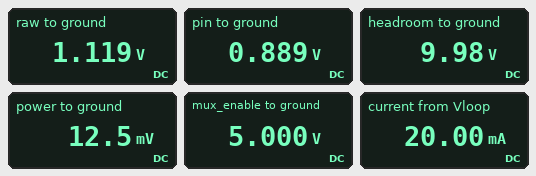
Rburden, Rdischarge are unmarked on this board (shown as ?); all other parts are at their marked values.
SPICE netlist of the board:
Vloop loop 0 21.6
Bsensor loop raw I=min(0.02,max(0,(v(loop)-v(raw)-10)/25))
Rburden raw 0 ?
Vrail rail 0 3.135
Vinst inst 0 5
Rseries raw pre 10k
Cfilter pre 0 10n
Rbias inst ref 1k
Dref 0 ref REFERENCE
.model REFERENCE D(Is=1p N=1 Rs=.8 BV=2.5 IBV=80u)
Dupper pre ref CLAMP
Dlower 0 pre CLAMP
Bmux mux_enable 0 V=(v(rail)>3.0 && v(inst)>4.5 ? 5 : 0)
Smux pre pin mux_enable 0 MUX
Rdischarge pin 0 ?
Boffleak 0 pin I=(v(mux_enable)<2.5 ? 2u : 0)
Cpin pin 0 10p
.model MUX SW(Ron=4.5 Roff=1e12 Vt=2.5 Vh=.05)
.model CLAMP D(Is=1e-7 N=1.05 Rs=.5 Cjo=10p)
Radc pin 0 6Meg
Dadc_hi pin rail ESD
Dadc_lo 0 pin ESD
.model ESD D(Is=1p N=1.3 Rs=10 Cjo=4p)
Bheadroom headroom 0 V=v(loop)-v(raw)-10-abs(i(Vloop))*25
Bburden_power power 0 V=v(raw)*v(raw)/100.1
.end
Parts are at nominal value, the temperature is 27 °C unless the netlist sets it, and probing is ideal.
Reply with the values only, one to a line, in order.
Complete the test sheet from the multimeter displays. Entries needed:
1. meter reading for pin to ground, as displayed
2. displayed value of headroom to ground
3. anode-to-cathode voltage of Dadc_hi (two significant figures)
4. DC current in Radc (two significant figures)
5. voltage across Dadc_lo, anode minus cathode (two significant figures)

0.889 V
9.98 V
-2.2 V
150 nA
-890 mV
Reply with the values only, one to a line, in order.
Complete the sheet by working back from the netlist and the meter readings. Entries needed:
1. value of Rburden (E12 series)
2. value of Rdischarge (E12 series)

56 Ω
39 kΩ
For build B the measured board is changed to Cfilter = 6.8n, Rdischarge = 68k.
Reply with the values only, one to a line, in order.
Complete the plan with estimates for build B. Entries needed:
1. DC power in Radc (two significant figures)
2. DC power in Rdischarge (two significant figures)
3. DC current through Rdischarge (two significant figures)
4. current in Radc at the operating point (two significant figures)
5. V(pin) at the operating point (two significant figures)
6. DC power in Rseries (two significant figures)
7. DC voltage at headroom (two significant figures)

160 nW
14 µW
14 µA
160 nA
970 mV
2.1 µW
10 V
